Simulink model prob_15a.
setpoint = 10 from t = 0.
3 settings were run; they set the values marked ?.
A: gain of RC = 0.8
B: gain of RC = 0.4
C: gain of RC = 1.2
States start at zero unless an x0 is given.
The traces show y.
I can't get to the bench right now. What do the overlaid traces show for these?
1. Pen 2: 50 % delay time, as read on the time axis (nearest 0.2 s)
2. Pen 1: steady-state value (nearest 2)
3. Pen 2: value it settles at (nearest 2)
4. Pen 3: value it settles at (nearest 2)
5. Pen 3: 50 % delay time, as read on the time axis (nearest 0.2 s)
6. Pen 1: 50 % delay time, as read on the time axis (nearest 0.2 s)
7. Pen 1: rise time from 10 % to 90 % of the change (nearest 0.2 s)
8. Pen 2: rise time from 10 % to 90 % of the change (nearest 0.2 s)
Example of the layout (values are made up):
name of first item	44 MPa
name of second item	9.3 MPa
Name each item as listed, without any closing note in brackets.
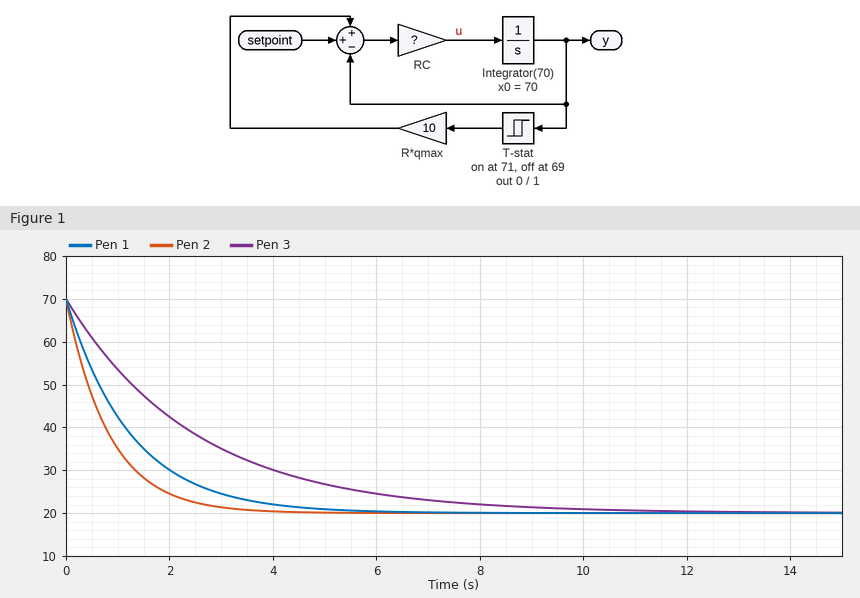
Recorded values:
Pen 2: 50 % delay time, as read on the time axis	0.6 s
Pen 1: steady-state value	20
Pen 2: value it settles at	20
Pen 3: value it settles at	20
Pen 3: 50 % delay time, as read on the time axis	1.8 s
Pen 1: 50 % delay time, as read on the time axis	0.8 s
Pen 1: rise time from 10 % to 90 % of the change	2.8 s
Pen 2: rise time from 10 % to 90 % of the change	1.8 s
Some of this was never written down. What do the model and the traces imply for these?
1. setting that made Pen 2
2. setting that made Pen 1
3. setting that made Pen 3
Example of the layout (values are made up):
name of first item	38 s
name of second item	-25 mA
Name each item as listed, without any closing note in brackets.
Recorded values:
setting that made Pen 2	C
setting that made Pen 1	A
setting that made Pen 3	B
